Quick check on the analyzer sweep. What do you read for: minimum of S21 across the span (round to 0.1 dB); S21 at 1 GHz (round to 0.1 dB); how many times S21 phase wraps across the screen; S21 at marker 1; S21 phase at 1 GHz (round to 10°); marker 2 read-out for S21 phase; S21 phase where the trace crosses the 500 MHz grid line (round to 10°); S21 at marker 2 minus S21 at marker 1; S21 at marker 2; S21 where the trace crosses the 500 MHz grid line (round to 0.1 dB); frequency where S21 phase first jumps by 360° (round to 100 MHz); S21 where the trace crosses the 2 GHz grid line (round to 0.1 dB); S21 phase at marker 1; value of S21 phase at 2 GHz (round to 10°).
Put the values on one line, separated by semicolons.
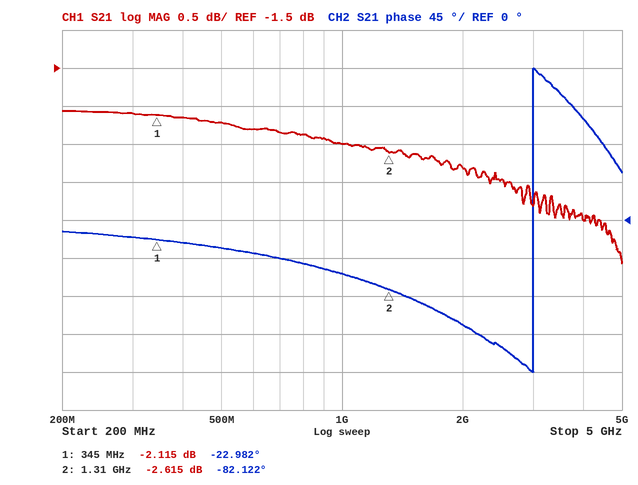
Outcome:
-4.1 dB; -2.5 dB; 1; -2.115 dB; -60°; -82.122°; -30°; -0.500 dB; -2.615 dB; -2.2 dB; 3.0 GHz; -2.8 dB; -22.982°; -120°
